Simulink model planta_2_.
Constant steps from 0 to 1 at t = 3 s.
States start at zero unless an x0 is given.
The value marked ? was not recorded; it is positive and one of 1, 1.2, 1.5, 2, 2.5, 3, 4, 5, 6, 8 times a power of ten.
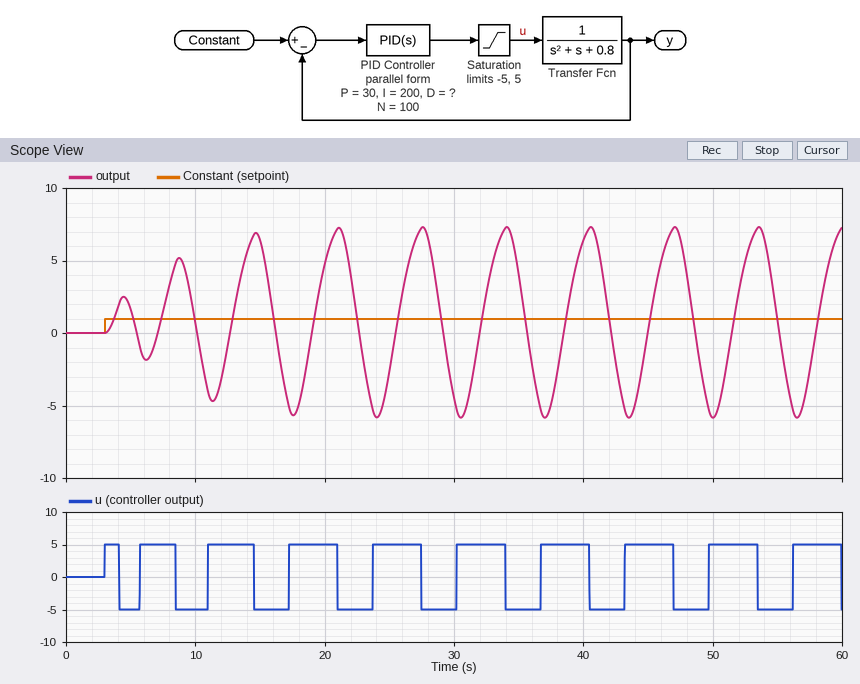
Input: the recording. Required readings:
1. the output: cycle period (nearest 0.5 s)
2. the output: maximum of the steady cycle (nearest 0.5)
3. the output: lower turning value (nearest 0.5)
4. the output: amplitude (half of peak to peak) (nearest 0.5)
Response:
6.5 s
7.5
-6.0
6.5
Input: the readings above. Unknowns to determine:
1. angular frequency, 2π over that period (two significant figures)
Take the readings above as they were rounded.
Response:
0.97 rad/s
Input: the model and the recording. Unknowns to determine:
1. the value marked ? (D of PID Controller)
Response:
8
